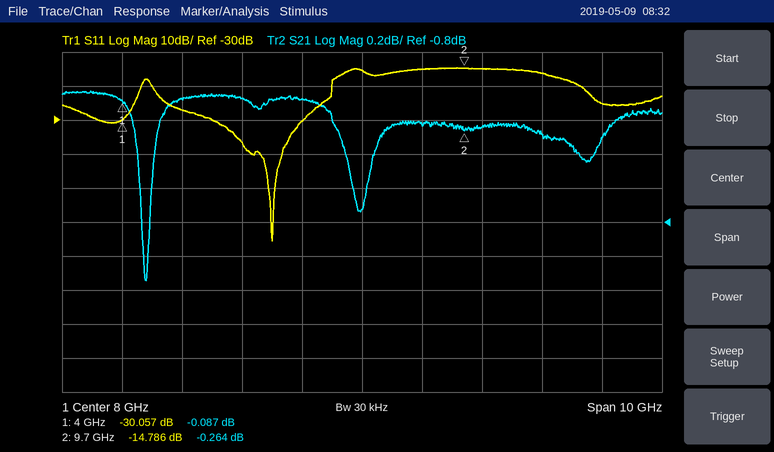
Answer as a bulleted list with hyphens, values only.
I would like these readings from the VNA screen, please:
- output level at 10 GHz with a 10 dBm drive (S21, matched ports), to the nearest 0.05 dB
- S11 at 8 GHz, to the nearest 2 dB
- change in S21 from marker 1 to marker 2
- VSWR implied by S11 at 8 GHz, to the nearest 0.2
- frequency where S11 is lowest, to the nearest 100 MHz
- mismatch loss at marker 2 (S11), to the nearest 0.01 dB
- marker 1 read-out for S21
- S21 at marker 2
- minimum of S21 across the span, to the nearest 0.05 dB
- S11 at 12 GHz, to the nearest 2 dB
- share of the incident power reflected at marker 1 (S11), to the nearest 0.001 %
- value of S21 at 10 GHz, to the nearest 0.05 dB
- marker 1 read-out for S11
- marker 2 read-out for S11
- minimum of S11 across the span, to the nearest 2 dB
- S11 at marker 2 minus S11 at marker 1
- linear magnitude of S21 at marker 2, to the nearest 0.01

- 9.75 dBm
- -16 dB
- -0.177 dB
- 1.4
- 6.5 GHz
- 0.15 dB
- -0.087 dB
- -0.264 dB
- -1.15 dB
- -26 dB
- 0.099 %
- -0.25 dB
- -30.057 dB
- -14.786 dB
- -66 dB
- 15.271 dB
- 0.97
